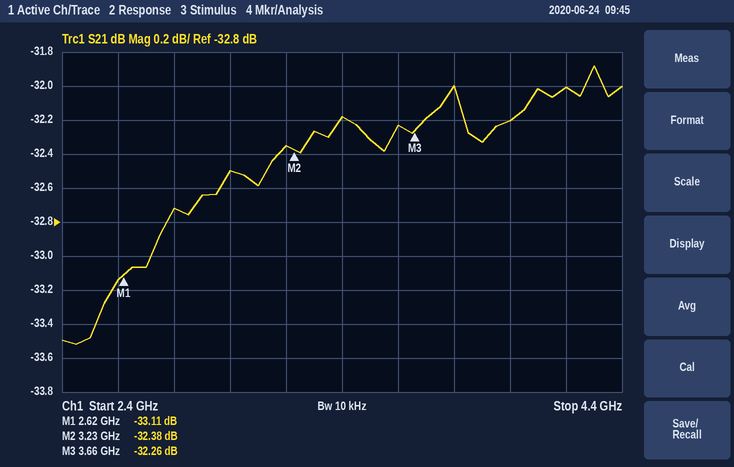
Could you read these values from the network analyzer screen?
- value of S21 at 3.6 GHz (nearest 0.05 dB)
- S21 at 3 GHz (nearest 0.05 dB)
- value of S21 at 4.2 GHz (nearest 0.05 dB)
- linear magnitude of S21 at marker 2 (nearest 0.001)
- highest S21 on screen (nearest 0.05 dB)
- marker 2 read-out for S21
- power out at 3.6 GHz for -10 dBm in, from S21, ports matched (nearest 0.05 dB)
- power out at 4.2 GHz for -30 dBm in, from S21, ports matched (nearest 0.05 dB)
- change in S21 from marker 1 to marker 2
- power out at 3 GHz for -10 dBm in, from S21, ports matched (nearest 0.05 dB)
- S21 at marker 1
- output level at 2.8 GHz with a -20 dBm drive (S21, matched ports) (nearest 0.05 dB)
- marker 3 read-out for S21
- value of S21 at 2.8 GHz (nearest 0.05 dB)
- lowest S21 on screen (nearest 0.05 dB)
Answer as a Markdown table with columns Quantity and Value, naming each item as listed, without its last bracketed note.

| Quantity | Value |
|---|---|
| value of S21 at 3.6 GHz | -32.25 dB |
| S21 at 3 GHz | -32.50 dB |
| value of S21 at 4.2 GHz | -32.00 dB |
| linear magnitude of S21 at marker 2 | 0.024 |
| highest S21 on screen | -31.90 dB |
| marker 2 read-out for S21 | -32.38 dB |
| power out at 3.6 GHz for -10 dBm in, from S21, ports matched | -42.25 dBm |
| power out at 4.2 GHz for -30 dBm in, from S21, ports matched | -62.00 dBm |
| change in S21 from marker 1 to marker 2 | 0.73 dB |
| power out at 3 GHz for -10 dBm in, from S21, ports matched | -42.50 dBm |
| S21 at marker 1 | -33.11 dB |
| output level at 2.8 GHz with a -20 dBm drive (S21, matched ports) | -52.70 dBm |
| marker 3 read-out for S21 | -32.26 dB |
| value of S21 at 2.8 GHz | -32.70 dB |
| lowest S21 on screen | -33.50 dB |
